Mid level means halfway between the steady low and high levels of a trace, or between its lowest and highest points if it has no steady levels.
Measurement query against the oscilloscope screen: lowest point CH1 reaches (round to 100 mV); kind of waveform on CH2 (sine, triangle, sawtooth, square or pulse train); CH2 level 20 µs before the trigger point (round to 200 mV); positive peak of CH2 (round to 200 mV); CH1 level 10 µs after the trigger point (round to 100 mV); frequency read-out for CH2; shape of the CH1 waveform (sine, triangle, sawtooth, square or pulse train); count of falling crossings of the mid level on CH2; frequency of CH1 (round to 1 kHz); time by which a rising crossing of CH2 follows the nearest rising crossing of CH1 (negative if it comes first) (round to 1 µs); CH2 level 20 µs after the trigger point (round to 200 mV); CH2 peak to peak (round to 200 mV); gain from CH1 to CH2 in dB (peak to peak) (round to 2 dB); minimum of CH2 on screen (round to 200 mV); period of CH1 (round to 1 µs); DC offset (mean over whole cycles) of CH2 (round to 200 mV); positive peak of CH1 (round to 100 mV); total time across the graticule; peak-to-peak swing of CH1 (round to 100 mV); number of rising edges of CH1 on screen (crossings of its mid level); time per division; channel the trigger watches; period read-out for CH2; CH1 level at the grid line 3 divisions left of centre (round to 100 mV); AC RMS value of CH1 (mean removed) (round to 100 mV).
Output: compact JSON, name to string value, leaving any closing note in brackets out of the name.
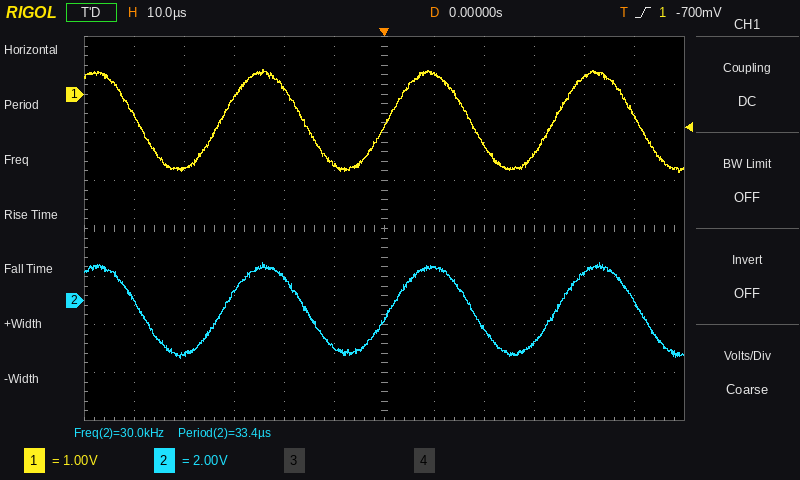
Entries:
{"lowest point CH1 reaches": "-1.6 V", "kind of waveform on CH2": "sine", "CH2 level 20 µs before the trigger point": "1.0 V", "positive peak of CH2": "1.6 V", "CH1 level 10 µs after the trigger point": "400 mV", "frequency read-out for CH2": "30.0 kHz", "shape of the CH1 waveform": "sine", "count of falling crossings of the mid level on CH2": "4", "frequency of CH1": "30 kHz", "time by which a rising crossing of CH2 follows the nearest rising crossing of CH1 (negative if it comes first)": "0 µs", "CH2 level 20 µs after the trigger point": "-1.2 V", "CH2 peak to peak": "4.0 V", "gain from CH1 to CH2 in dB (peak to peak)": "6 dB", "minimum of CH2 on screen": "-2.4 V", "period of CH1": "33 µs", "DC offset (mean over whole cycles) of CH2": "-400 mV", "positive peak of CH1": "500 mV", "total time across the graticule": "120 µs", "peak-to-peak swing of CH1": "2.1 V", "number of rising edges of CH1 on screen": "3", "time per division": "10 µs", "channel the trigger watches": "CH1", "period read-out for CH2": "33.4 µs", "CH1 level at the grid line 3 divisions left of centre": "-100 mV", "AC RMS value of CH1 (mean removed)": "700 mV"}
